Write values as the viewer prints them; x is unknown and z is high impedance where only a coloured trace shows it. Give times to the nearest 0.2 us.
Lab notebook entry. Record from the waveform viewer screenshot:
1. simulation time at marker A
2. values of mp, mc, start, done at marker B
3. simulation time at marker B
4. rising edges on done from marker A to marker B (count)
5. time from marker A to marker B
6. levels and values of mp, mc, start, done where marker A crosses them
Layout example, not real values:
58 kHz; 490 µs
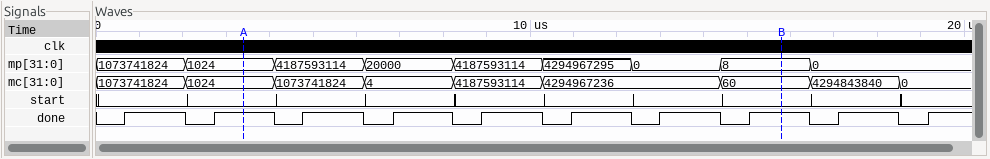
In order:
3.4 us; mp=8, mc=60, start=0, done=1; 15.8 us; 6; 12.4 us; mp=1024, mc=1024, start=0, done=1
